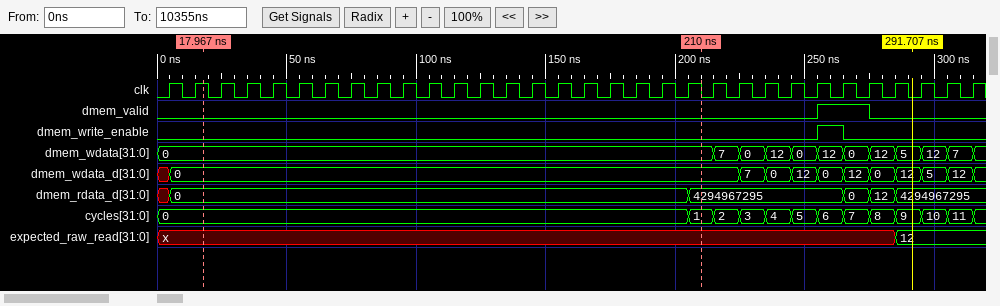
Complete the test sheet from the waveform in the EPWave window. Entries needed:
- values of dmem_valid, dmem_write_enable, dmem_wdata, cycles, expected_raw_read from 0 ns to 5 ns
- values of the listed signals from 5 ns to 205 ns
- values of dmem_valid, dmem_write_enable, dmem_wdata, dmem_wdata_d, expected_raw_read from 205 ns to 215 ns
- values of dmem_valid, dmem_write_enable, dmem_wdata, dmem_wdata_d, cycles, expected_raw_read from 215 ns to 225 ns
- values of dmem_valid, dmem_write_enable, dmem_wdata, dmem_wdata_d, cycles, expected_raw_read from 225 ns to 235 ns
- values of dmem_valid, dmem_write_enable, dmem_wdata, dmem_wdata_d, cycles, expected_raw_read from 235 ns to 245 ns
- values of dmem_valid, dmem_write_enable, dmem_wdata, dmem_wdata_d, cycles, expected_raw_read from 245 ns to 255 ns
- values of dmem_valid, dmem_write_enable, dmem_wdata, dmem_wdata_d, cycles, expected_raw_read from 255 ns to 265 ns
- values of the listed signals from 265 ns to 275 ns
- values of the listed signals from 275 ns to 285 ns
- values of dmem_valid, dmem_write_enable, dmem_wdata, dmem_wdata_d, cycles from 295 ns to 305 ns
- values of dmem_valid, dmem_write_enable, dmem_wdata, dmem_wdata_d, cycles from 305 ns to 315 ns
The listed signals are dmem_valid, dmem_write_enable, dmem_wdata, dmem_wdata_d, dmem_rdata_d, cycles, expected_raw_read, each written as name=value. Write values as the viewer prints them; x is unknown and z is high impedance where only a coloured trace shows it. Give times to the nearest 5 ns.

dmem_valid=0, dmem_write_enable=0, dmem_wdata=0, cycles=0, expected_raw_read=x
dmem_valid=0, dmem_write_enable=0, dmem_wdata=0, dmem_wdata_d=0, dmem_rdata_d=0, cycles=0, expected_raw_read=x
dmem_valid=0, dmem_write_enable=0, dmem_wdata=0, dmem_wdata_d=0, expected_raw_read=x
dmem_valid=0, dmem_write_enable=0, dmem_wdata=7, dmem_wdata_d=0, cycles=2, expected_raw_read=x
dmem_valid=0, dmem_write_enable=0, dmem_wdata=0, dmem_wdata_d=7, cycles=3, expected_raw_read=x
dmem_valid=0, dmem_write_enable=0, dmem_wdata=12, dmem_wdata_d=0, cycles=4, expected_raw_read=x
dmem_valid=0, dmem_write_enable=0, dmem_wdata=0, dmem_wdata_d=12, cycles=5, expected_raw_read=x
dmem_valid=1, dmem_write_enable=1, dmem_wdata=12, dmem_wdata_d=0, cycles=6, expected_raw_read=x
dmem_valid=1, dmem_write_enable=0, dmem_wdata=0, dmem_wdata_d=12, dmem_rdata_d=0, cycles=7, expected_raw_read=x
dmem_valid=0, dmem_write_enable=0, dmem_wdata=12, dmem_wdata_d=0, dmem_rdata_d=12, cycles=8, expected_raw_read=x
dmem_valid=0, dmem_write_enable=0, dmem_wdata=12, dmem_wdata_d=5, cycles=10
dmem_valid=0, dmem_write_enable=0, dmem_wdata=7, dmem_wdata_d=12, cycles=11
